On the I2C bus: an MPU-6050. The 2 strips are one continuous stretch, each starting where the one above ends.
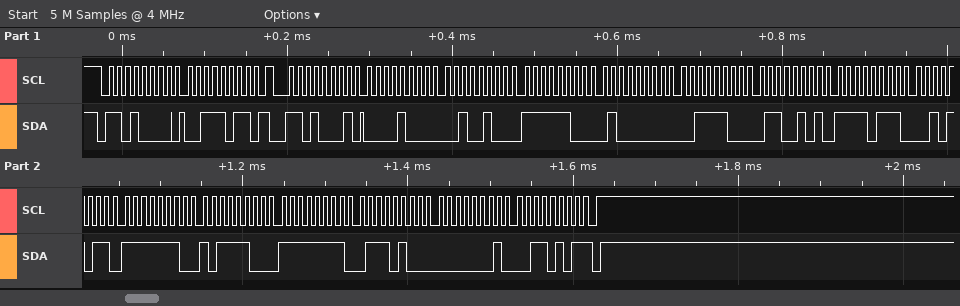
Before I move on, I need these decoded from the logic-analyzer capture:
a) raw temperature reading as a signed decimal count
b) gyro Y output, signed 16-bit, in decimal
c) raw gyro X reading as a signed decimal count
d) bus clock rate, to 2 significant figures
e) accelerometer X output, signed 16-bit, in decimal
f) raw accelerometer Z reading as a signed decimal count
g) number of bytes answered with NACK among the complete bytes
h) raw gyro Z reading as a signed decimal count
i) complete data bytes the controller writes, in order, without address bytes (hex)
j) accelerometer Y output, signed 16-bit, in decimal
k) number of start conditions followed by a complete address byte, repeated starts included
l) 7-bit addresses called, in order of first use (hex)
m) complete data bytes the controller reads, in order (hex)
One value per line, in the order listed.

-2261
-140
-324
100 kHz
2084
15461
1
309
3B
-960
2
0x68
08 24 FC 40 3C 65 F7 2B FE BC FF 74 01 35
